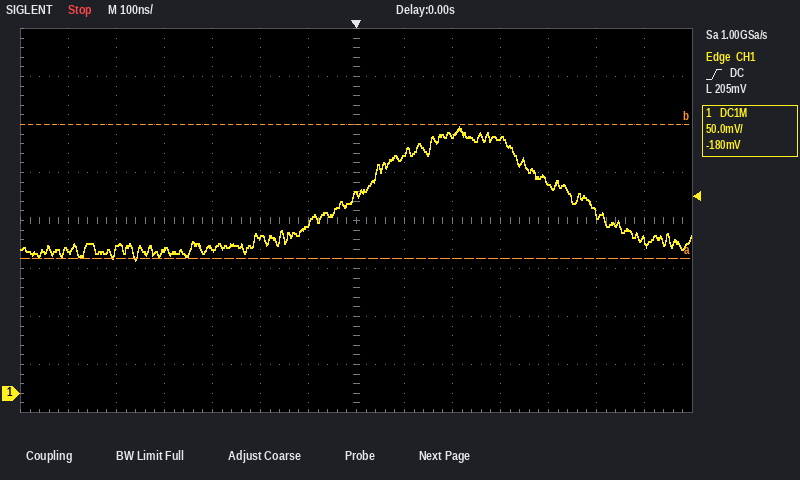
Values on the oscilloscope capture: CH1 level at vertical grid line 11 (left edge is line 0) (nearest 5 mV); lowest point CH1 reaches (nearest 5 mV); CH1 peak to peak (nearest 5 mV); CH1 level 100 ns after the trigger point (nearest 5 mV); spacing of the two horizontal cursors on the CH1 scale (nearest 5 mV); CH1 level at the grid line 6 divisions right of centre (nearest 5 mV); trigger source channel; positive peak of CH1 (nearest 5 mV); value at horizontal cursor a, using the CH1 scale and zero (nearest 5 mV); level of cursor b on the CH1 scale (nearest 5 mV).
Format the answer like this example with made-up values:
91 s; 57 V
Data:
220 mV; 140 mV; 140 mV; 250 mV; 140 mV; 160 mV; CH1; 280 mV; 140 mV; 280 mV
